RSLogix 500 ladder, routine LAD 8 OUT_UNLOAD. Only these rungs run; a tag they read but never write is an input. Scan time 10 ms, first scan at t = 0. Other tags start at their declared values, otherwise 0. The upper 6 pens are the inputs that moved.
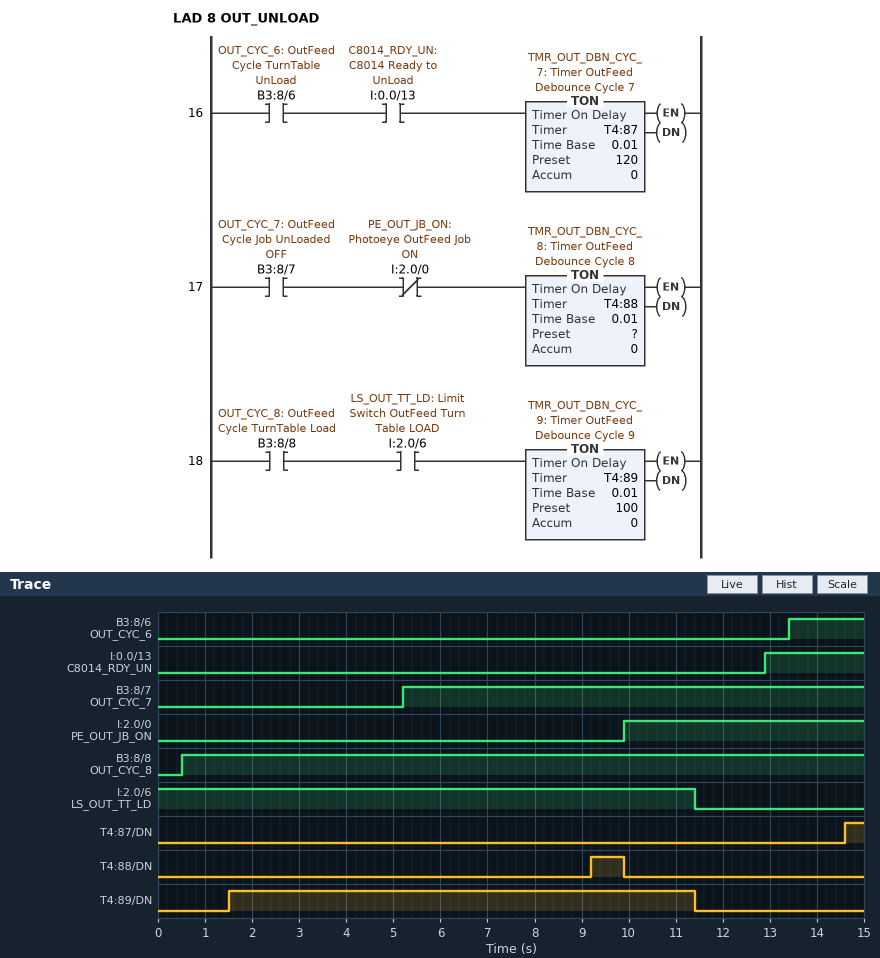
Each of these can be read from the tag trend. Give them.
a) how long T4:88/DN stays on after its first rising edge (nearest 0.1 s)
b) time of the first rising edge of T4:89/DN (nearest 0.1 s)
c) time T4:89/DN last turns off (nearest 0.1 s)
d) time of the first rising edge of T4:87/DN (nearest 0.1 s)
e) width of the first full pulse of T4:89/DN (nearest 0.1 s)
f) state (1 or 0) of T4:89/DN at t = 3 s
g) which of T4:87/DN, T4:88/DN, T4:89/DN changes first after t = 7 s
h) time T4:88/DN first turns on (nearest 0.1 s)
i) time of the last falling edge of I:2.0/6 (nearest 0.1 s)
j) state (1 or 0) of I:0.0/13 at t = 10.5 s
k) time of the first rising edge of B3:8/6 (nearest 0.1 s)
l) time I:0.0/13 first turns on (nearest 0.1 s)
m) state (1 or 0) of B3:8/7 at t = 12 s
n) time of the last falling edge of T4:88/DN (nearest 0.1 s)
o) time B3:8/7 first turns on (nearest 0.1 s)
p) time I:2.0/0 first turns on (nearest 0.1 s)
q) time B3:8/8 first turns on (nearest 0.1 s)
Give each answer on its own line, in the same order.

0.7 s
1.5 s
11.4 s
14.6 s
9.9 s
1
T4:88/DN
9.2 s
11.4 s
0
13.4 s
12.9 s
1
9.9 s
5.2 s
9.9 s
0.5 s
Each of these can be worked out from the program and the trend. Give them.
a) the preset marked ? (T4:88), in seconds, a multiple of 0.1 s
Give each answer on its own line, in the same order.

4.0 s
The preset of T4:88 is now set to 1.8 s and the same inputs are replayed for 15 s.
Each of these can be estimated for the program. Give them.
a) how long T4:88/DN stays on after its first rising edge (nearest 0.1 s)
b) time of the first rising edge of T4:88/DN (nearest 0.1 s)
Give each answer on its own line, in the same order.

2.9 s
7.0 s
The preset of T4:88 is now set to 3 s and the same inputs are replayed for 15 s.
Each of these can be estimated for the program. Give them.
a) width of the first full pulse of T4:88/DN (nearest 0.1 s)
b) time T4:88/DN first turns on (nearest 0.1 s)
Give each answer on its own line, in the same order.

1.7 s
8.2 s
